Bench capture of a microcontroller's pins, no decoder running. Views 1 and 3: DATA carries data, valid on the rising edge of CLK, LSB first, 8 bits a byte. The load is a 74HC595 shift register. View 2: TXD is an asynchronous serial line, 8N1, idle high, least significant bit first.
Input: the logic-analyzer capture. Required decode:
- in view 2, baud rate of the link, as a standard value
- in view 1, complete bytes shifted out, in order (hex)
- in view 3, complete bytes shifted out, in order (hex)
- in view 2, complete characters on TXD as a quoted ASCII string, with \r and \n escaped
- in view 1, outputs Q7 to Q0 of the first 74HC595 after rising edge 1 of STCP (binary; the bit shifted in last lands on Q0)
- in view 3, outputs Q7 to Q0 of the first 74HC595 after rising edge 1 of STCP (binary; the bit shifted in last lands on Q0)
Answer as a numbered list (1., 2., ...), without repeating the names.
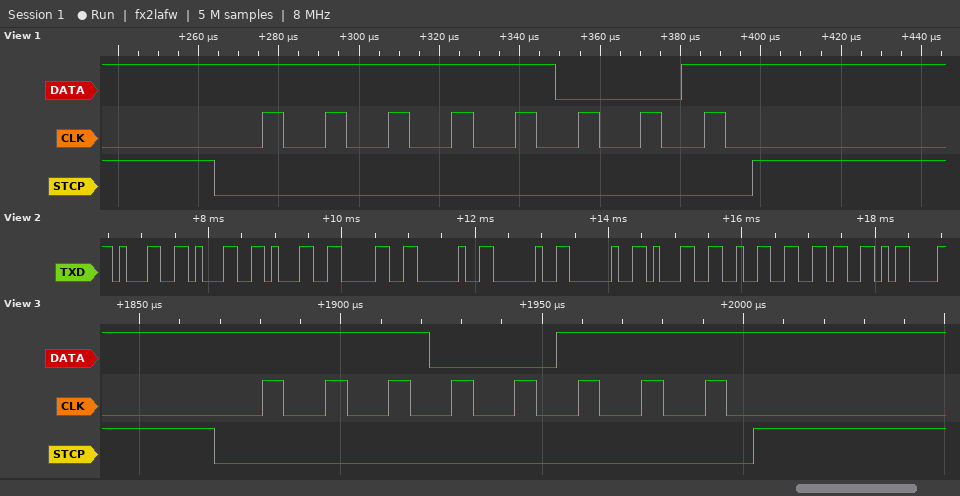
1. 9600 baud
2. 9F
3. 0xE7
4. "1110   126\r"
5. 11111001
6. 11100111
